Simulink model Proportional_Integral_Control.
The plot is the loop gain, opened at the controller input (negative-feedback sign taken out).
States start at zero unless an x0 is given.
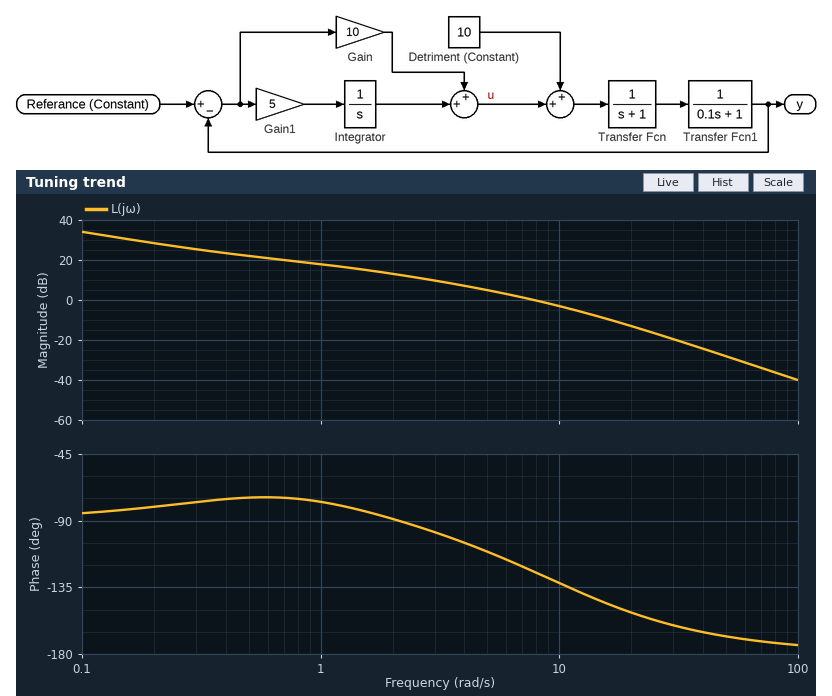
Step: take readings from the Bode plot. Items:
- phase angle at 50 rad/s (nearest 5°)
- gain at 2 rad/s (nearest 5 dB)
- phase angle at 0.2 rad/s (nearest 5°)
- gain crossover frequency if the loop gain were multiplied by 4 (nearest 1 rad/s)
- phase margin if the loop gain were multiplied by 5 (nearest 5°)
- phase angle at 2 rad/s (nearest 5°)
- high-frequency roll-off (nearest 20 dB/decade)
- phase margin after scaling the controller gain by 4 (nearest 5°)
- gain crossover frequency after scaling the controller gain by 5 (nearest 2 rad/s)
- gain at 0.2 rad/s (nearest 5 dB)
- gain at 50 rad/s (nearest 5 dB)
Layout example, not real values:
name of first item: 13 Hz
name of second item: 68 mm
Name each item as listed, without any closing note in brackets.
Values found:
phase angle at 50 rad/s: -170°
gain at 2 rad/s: 15 dB
phase angle at 0.2 rad/s: -80°
gain crossover frequency if the loop gain were multiplied by 4: 19 rad/s
phase margin if the loop gain were multiplied by 5: 25°
phase angle at 2 rad/s: -90°
high-frequency roll-off: -40 dB/decade
phase margin after scaling the controller gain by 4: 30°
gain crossover frequency after scaling the controller gain by 5: 22 rad/s
gain at 0.2 rad/s: 30 dB
gain at 50 rad/s: -30 dB
